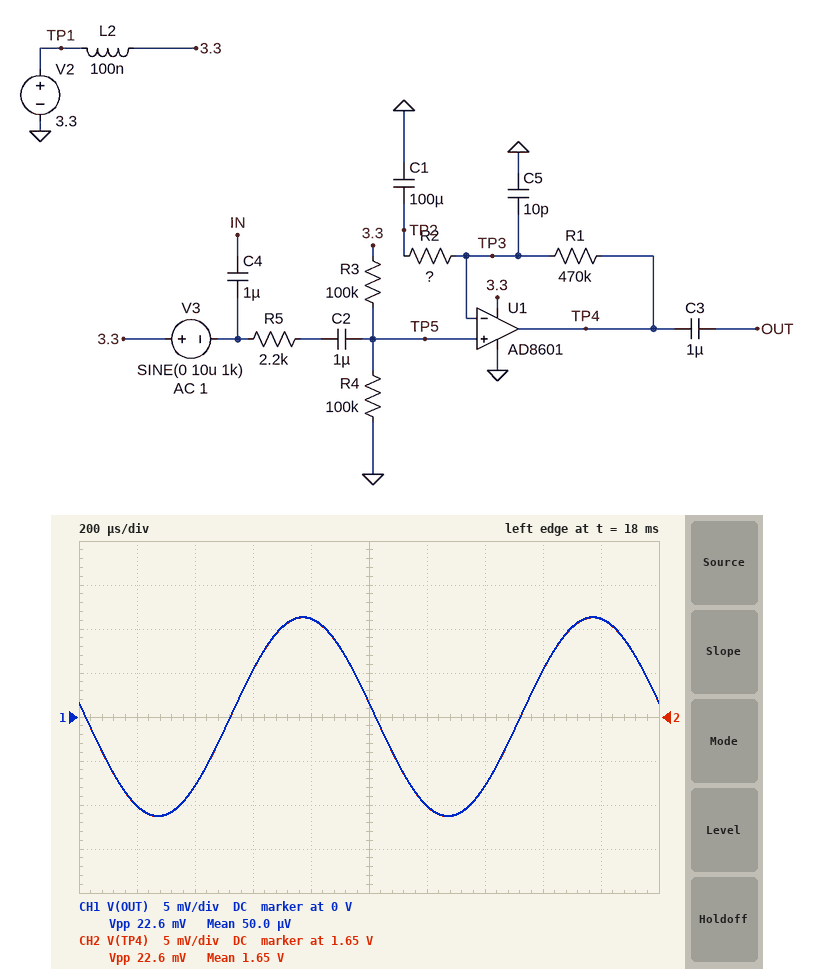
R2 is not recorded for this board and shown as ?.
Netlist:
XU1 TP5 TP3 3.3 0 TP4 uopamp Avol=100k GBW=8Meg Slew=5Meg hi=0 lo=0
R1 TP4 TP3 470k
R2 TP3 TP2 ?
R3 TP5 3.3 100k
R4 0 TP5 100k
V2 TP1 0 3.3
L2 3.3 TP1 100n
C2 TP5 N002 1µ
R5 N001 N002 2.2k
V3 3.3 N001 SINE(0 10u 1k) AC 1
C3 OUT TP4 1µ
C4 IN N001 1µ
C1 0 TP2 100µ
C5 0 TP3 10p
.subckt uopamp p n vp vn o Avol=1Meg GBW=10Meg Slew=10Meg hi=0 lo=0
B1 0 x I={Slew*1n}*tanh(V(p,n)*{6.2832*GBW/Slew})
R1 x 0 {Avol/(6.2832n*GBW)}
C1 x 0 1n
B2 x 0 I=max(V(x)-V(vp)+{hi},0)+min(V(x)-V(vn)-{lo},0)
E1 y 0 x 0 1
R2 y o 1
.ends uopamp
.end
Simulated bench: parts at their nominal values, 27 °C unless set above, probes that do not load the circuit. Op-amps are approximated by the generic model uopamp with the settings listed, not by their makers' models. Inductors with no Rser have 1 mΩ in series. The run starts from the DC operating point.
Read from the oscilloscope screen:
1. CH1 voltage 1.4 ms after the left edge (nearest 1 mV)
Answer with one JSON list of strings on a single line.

["-8 mV"]
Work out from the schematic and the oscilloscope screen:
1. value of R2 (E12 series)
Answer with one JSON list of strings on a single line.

["390 Ω"]
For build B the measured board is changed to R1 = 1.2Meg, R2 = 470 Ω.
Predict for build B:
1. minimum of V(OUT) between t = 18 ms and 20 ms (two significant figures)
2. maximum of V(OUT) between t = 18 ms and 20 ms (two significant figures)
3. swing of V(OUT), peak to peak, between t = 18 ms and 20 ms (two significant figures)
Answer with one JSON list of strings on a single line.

["-23 mV", "23 mV", "46 mV"]
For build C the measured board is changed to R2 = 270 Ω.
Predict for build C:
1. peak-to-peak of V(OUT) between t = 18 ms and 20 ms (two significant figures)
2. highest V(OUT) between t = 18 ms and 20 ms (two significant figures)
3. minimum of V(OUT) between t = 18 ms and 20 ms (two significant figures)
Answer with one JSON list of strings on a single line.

["32 mV", "16 mV", "-16 mV"]
